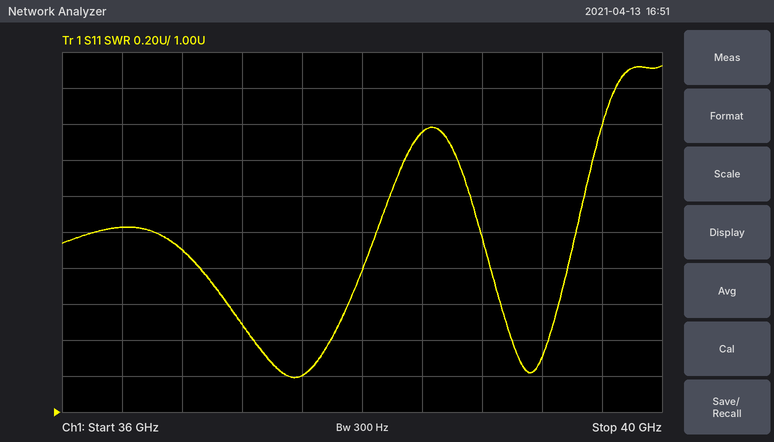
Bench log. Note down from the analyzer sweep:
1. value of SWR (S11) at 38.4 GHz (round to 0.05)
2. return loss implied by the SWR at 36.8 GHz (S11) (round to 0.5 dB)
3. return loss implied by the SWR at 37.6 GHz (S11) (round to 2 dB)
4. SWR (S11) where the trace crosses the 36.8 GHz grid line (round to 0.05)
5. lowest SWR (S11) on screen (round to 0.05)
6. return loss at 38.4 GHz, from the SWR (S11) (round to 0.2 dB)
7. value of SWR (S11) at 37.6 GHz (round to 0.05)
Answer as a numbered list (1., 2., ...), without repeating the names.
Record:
1. 2.55
2. 10.0 dB
3. 20 dB
4. 1.90
5. 1.20
6. 7.2 dB
7. 1.20
